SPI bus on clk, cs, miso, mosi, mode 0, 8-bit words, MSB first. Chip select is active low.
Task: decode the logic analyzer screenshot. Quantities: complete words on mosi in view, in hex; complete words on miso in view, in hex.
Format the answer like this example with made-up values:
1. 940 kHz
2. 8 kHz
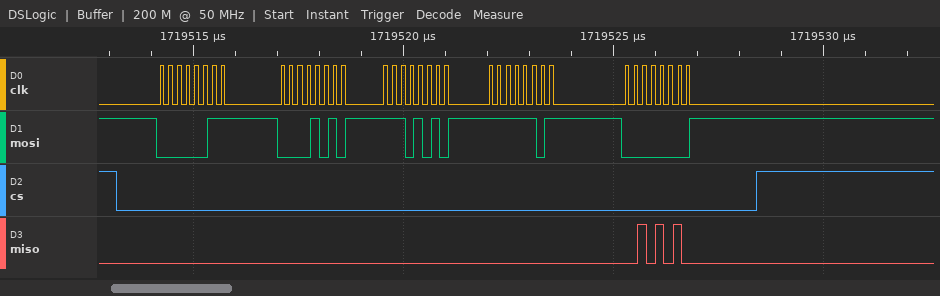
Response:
1. 03, 0A, EA, FD, 00
2. 00, 00, 00, 00, 2A
